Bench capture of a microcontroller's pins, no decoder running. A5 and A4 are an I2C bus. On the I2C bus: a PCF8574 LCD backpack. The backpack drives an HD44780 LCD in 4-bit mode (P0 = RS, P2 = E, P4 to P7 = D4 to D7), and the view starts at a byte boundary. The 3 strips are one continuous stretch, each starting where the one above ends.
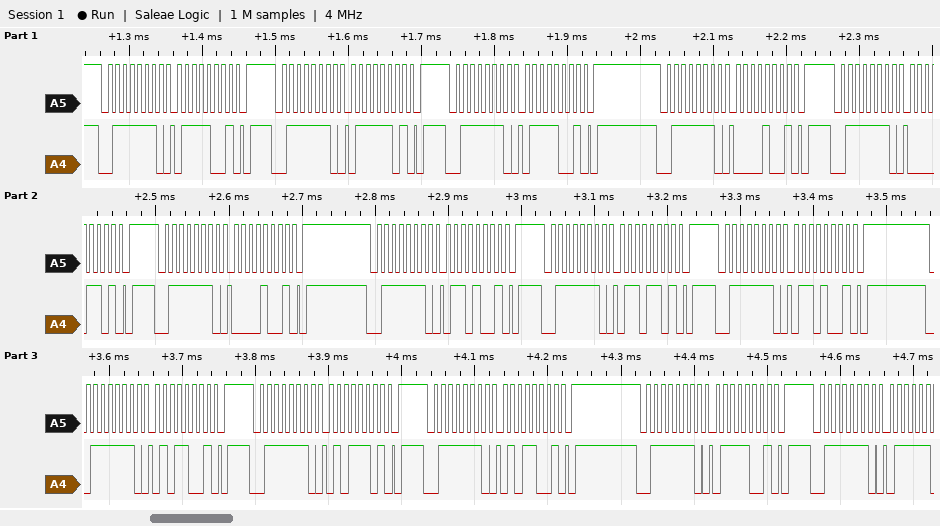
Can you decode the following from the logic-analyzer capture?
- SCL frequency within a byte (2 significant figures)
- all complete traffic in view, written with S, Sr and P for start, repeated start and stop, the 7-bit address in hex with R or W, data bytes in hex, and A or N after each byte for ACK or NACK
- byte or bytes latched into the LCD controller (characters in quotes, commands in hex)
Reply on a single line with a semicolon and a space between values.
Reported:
100 kHz; S 3FW A 79 A P S 3FW A 7D A P S 3FW A 79 A P S 3FW A 09 A P S 3FW A 0D A P S 3FW A 09 A P S 3FW A 69 A P S 3FW A 6D A P S 3FW A 69 A P S 3FW A 59 A P S 3FW A 5D A P S 3FW A 59 A P S 3FW A 79 A P S 3FW A; 'p' 'e'
